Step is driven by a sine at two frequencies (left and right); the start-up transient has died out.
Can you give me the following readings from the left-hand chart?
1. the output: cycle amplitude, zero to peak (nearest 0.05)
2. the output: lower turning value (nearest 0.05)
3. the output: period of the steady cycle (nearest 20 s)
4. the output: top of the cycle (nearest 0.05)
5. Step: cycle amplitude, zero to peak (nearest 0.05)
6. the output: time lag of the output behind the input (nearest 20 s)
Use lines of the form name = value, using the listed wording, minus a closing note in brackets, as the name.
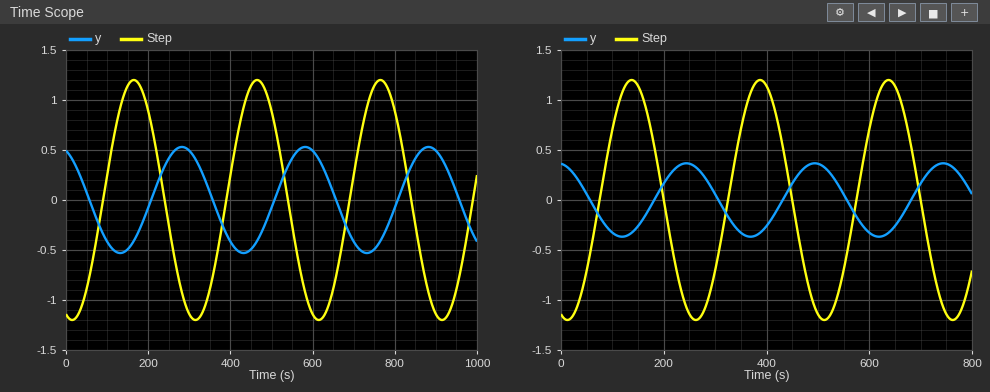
the output: cycle amplitude, zero to peak = 0.55
the output: lower turning value = -0.55
the output: period of the steady cycle = 300 s
the output: top of the cycle = 0.55
Step: cycle amplitude, zero to peak = 1.20
the output: time lag of the output behind the input = 120 s
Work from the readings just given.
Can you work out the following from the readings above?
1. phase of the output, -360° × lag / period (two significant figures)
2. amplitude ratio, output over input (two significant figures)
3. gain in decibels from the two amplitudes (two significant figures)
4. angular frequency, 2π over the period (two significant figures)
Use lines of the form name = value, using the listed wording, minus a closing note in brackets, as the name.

phase of the output, -360° × lag / period = -140°
amplitude ratio, output over input = 0.46
gain in decibels from the two amplitudes = -6.8 dB
angular frequency, 2π over the period = 0.021 rad/s
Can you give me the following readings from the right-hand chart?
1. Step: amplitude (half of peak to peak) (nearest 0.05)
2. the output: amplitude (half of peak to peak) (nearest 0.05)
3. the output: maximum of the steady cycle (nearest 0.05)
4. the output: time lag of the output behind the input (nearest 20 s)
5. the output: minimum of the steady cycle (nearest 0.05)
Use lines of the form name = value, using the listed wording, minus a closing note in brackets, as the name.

Step: amplitude (half of peak to peak) = 1.20
the output: amplitude (half of peak to peak) = 0.35
the output: maximum of the steady cycle = 0.35
the output: time lag of the output behind the input = 100 s
the output: minimum of the steady cycle = -0.35
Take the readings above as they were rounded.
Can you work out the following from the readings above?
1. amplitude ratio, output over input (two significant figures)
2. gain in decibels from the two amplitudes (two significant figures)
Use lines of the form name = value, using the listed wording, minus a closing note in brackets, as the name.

amplitude ratio, output over input = 0.29
gain in decibels from the two amplitudes = -11 dB
